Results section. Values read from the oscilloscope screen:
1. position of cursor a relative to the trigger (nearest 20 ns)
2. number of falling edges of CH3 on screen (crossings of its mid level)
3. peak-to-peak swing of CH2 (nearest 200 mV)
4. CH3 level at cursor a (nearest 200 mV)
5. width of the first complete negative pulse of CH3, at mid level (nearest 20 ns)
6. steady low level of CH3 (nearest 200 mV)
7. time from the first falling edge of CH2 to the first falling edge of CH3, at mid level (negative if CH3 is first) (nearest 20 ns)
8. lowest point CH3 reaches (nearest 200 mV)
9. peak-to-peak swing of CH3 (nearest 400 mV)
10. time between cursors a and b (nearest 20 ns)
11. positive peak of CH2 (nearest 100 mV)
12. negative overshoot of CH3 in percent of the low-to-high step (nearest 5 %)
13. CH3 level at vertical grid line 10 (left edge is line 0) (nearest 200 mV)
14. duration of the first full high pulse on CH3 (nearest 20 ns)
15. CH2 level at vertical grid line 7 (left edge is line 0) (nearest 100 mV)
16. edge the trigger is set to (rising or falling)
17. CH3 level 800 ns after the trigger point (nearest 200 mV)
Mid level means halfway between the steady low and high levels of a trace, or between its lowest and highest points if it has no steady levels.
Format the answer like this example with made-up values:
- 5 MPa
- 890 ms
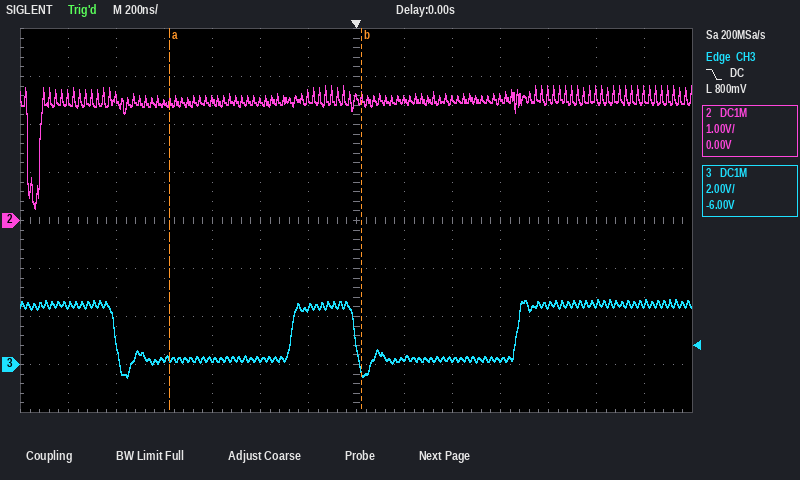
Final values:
- -780 ns
- 2
- 2.6 V
- 200 mV
- 740 ns
- 200 mV
- +360 ns
- -600 mV
- 3.2 V
- 800 ns
- 2.8 V
- 35 %
- 200 mV
- 260 ns
- 2.6 V
- falling
- 2.4 V
